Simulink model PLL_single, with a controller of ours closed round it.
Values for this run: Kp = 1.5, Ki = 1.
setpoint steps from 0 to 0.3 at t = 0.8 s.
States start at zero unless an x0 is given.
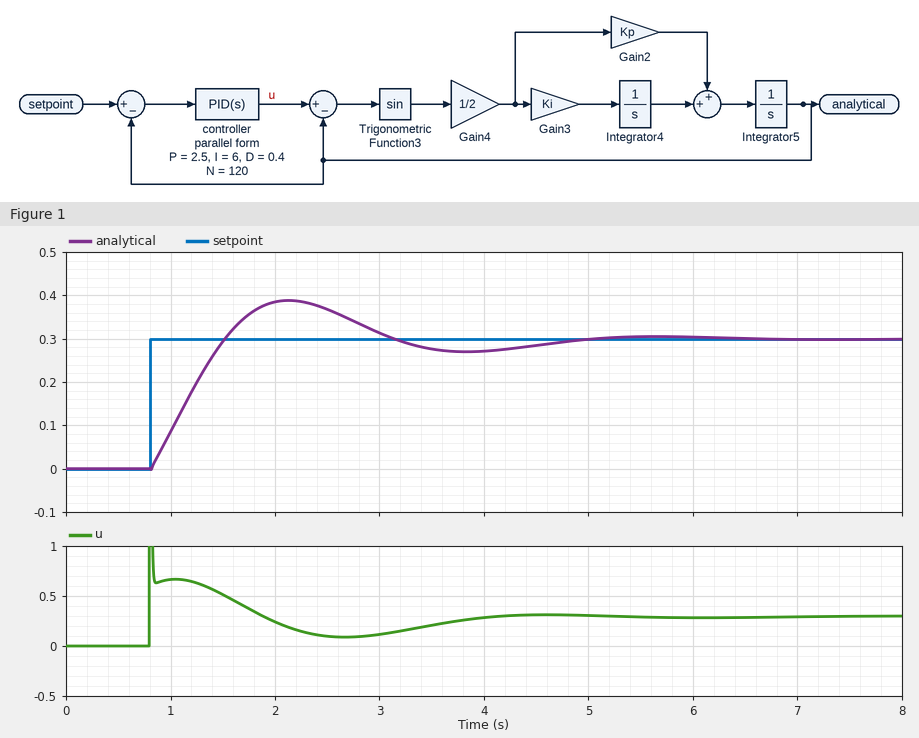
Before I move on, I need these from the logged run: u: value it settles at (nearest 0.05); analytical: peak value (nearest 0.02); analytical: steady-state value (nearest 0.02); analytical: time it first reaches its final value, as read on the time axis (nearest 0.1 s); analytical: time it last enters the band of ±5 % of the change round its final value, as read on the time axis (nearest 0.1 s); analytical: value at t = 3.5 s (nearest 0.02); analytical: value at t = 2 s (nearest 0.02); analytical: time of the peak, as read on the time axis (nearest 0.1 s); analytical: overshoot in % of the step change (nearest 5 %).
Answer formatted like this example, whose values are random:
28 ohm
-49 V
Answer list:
0.30
0.38
0.30
1.5 s
4.5 s
0.28
0.38
2.1 s
30 %
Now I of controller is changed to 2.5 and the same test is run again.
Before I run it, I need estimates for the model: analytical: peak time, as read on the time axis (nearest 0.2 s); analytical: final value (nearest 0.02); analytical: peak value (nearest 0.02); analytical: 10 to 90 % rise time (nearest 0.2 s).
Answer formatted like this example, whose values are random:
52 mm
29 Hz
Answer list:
2.6 s
0.30
0.34
0.8 s
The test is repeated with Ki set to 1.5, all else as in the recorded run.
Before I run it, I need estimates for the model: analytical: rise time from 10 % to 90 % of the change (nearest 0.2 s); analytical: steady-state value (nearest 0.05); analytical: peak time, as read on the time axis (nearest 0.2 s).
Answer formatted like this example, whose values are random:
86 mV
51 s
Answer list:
0.6 s
0.30
2.0 s
